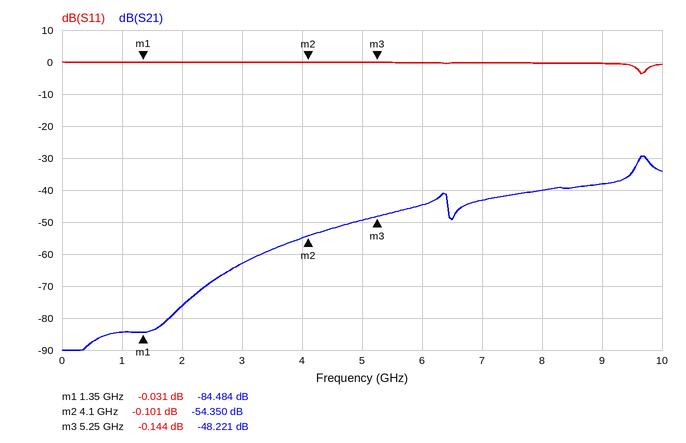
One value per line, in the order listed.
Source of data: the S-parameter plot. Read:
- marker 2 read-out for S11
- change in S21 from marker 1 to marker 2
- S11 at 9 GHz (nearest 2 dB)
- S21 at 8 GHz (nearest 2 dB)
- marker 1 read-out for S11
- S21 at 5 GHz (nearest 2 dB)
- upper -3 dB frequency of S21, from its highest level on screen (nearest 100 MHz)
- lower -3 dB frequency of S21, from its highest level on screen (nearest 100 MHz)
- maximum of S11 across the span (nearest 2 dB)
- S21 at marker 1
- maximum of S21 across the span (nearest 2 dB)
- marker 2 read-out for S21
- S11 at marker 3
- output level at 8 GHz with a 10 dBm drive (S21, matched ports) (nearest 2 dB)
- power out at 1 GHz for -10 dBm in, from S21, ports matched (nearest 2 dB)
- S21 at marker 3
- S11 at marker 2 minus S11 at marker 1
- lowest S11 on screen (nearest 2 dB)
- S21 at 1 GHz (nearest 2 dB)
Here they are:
-0.101 dB
30.134 dB
0 dB
-40 dB
-0.031 dB
-50 dB
9.8 GHz
9.6 GHz
0 dB
-84.484 dB
-30 dB
-54.350 dB
-0.144 dB
-30 dBm
-94 dBm
-48.221 dB
-0.070 dB
-4 dB
-84 dB
